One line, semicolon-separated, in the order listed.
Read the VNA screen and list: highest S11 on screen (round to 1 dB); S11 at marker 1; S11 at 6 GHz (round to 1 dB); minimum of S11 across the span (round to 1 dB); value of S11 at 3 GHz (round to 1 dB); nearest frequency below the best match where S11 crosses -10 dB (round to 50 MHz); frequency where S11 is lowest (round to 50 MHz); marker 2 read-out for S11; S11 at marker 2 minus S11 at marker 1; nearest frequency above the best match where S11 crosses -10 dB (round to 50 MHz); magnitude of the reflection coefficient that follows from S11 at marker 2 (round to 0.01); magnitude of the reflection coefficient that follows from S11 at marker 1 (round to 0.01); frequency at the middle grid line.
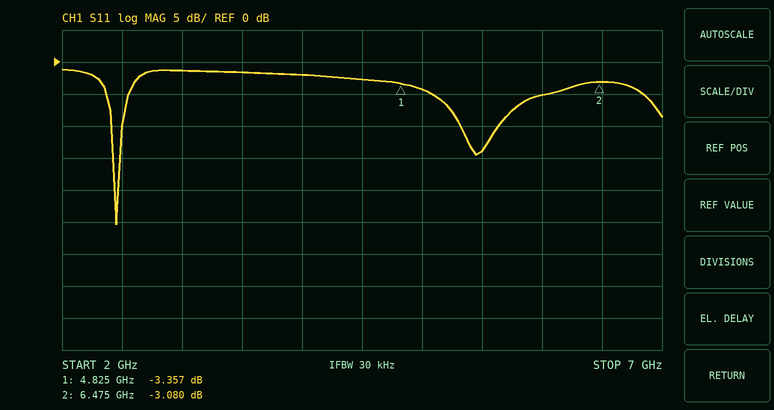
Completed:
-1 dB; -3.357 dB; -5 dB; -25 dB; -1 dB; 2.40 GHz; 2.45 GHz; -3.080 dB; 0.277 dB; 2.50 GHz; 0.70; 0.68; 4.5 GHz
